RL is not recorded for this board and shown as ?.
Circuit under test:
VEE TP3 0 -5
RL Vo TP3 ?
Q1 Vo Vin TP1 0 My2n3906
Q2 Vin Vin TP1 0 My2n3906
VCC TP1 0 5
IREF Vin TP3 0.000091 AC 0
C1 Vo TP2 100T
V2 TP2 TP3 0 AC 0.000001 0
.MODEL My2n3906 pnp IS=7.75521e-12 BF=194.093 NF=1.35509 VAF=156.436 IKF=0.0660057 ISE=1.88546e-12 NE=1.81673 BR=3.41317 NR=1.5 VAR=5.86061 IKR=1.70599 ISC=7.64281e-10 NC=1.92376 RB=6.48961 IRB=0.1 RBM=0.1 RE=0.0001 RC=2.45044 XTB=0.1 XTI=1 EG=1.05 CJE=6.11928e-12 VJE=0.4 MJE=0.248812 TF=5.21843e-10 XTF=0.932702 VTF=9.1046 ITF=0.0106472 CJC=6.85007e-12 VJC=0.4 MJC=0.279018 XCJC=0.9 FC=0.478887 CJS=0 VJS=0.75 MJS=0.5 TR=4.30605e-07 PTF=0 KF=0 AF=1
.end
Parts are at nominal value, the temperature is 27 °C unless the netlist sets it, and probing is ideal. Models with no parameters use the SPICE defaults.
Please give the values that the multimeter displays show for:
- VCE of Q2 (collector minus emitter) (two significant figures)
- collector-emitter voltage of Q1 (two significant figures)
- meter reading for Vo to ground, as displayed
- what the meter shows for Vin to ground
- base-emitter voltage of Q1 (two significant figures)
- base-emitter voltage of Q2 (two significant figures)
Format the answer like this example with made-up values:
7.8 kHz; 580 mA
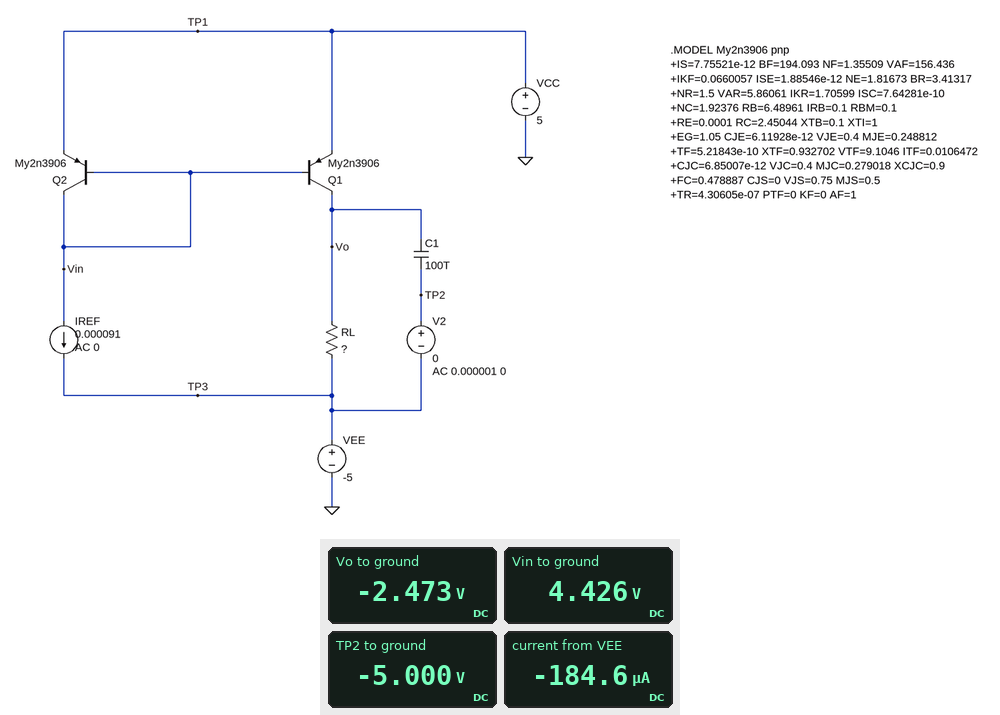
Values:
-570 mV; -7.5 V; -2.473 V; 4.426 V; -570 mV; -570 mV
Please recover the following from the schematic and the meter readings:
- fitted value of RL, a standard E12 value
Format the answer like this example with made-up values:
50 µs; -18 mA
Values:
27 kΩ
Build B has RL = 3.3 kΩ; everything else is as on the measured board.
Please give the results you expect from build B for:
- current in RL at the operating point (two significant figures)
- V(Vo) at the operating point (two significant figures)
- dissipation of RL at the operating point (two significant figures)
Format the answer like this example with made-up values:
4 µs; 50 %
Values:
95 µA; -4.7 V; 30 µW
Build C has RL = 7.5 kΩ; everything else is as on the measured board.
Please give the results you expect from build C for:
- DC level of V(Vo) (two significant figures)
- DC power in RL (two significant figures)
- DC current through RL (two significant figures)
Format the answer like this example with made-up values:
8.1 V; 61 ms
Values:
-4.3 V; 67 µW; 95 µA
